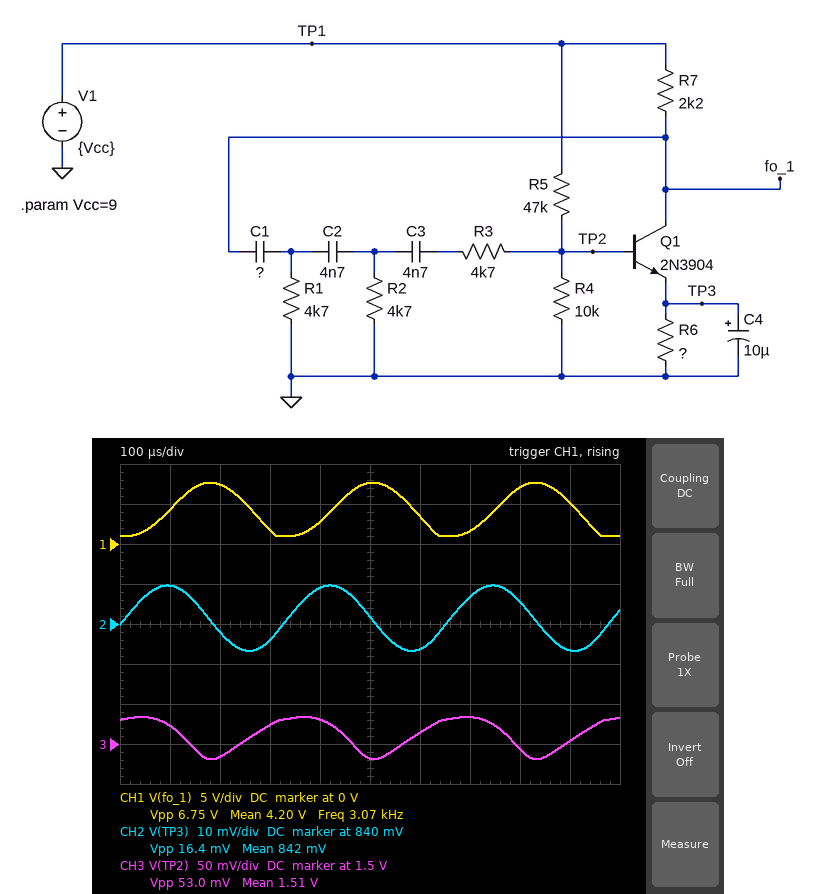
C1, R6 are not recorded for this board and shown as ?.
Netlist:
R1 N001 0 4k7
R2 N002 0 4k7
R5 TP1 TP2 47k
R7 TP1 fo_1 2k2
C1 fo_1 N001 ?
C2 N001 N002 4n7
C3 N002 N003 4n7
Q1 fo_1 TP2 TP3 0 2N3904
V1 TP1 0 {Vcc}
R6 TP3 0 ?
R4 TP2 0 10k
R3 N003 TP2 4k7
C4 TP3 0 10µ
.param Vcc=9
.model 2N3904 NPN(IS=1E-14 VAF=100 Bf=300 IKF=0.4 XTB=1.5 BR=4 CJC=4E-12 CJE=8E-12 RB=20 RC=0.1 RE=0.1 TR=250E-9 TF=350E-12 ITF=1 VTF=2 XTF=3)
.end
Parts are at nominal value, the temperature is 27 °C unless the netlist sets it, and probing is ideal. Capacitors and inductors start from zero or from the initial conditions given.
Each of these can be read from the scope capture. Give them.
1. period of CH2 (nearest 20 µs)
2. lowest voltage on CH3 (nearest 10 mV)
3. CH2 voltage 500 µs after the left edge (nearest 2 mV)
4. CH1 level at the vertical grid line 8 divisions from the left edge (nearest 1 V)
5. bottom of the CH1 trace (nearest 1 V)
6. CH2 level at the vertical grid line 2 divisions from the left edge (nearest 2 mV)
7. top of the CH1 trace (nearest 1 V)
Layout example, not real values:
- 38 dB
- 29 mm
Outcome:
- 320 µs
- 1.48 V
- 842 mV
- 7 V
- 1 V
- 838 mV
- 8 V
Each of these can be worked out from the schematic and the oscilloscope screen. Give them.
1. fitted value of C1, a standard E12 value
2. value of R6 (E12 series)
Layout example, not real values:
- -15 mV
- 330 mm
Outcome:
- 1.8 nF
- 390 Ω
